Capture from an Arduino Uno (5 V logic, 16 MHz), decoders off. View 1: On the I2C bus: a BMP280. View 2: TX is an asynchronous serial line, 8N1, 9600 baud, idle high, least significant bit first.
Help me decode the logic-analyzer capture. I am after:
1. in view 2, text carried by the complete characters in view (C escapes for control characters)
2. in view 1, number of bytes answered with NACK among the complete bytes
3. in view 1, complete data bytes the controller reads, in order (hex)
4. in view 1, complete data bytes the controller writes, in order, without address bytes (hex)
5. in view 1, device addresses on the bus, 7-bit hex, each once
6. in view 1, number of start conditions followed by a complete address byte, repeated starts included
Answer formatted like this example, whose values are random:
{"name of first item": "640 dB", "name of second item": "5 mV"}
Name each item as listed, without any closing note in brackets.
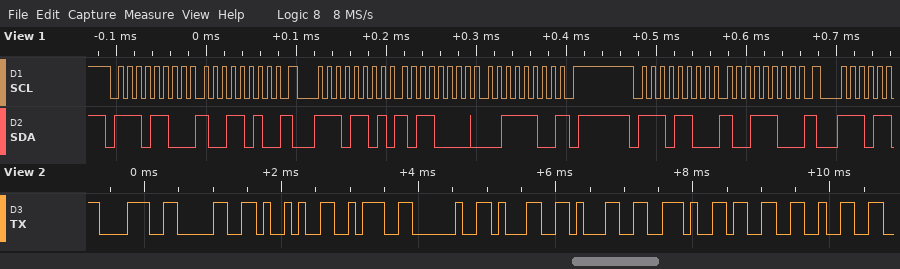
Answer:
{"in view 2, text carried by the complete characters in view": "\"80): 11.32\"", "in view 1, number of bytes answered with NACK among the complete bytes": "1", "in view 1, complete data bytes the controller reads, in order": "B0 3C", "in view 1, complete data bytes the controller writes, in order, without address bytes": "9A 9C", "in view 1, device addresses on the bus, 7-bit hex, each once": "0x76", "in view 1, number of start conditions followed by a complete address byte, repeated starts included": "3"}
